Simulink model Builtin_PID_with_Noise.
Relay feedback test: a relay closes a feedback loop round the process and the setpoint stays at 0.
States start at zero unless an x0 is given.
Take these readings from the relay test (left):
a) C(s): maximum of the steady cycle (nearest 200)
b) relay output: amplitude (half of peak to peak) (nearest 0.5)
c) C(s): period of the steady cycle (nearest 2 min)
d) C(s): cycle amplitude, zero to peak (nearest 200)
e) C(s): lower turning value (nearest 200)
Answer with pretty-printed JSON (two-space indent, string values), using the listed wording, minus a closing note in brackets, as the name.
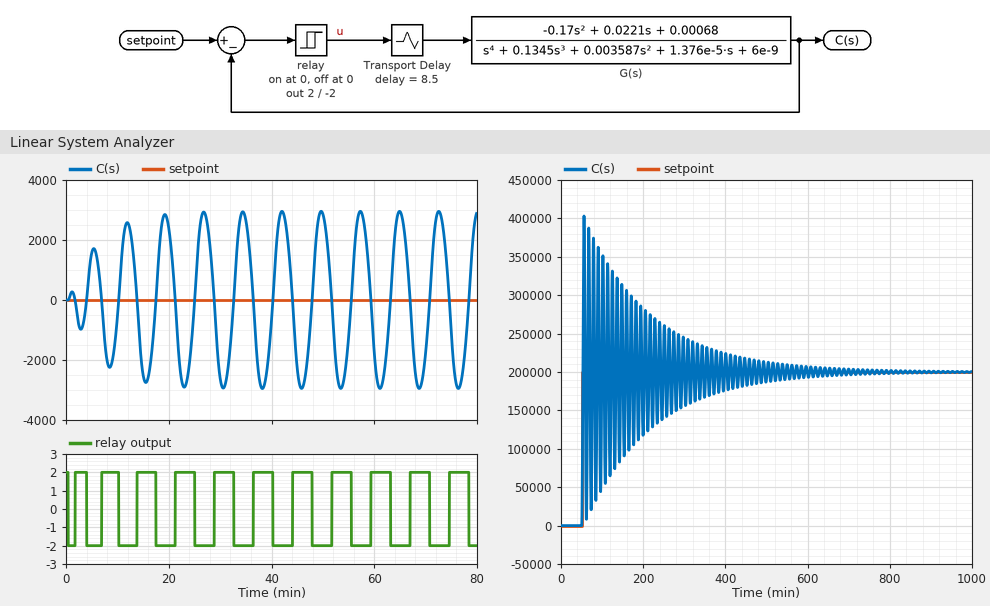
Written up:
{
  "C(s): maximum of the steady cycle": "3000",
  "relay output: amplitude (half of peak to peak)": "2.0",
  "C(s): period of the steady cycle": "8 min",
  "C(s): cycle amplitude, zero to peak": "3000",
  "C(s): lower turning value": "-3000"
}
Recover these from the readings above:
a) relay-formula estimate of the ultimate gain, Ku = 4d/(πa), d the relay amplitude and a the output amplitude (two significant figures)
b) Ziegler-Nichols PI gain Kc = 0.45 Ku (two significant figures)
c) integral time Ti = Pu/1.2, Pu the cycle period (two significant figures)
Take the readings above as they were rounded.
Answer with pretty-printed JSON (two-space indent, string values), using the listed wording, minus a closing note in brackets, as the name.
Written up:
{
  "relay-formula estimate of the ultimate gain, Ku = 4d/(πa), d the relay amplitude and a the output amplitude": "0.00085",
  "Ziegler-Nichols PI gain Kc = 0.45 Ku": "0.00038",
  "integral time Ti = Pu/1.2, Pu the cycle period": "6.7 min"
}
